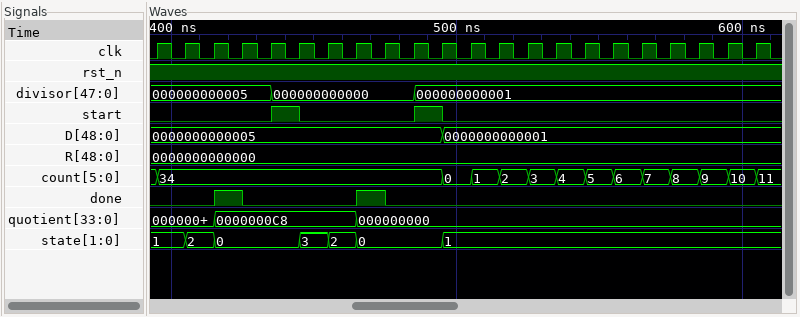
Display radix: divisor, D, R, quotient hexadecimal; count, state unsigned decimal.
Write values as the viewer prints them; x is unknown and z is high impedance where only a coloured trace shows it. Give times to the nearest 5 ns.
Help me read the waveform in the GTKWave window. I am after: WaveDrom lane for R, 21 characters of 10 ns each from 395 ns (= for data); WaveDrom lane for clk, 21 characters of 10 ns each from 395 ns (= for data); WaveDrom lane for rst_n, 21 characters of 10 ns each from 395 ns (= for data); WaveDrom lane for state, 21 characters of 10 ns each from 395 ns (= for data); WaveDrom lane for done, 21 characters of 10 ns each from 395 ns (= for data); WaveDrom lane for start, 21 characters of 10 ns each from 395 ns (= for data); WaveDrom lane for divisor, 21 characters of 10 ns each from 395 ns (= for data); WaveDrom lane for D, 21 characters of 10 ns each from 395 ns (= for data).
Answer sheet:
{name: 'R', wave: '=....................', data: '0000000000000'}
{name: 'clk', wave: 'p....................'}
{name: 'rst_n', wave: '1....................'}
{name: 'state', wave: '===..===..=..........', data: '1 2 0 3 2 0 1'}
{name: 'done', wave: '0.10...10............'}
{name: 'start', wave: '0...10...10..........'}
{name: 'divisor', wave: '=...=....=...........', data: '000000000005 000000000000 000000000001'}
{name: 'D', wave: '=.........=..........', data: '0000000000005 0000000000001'}
